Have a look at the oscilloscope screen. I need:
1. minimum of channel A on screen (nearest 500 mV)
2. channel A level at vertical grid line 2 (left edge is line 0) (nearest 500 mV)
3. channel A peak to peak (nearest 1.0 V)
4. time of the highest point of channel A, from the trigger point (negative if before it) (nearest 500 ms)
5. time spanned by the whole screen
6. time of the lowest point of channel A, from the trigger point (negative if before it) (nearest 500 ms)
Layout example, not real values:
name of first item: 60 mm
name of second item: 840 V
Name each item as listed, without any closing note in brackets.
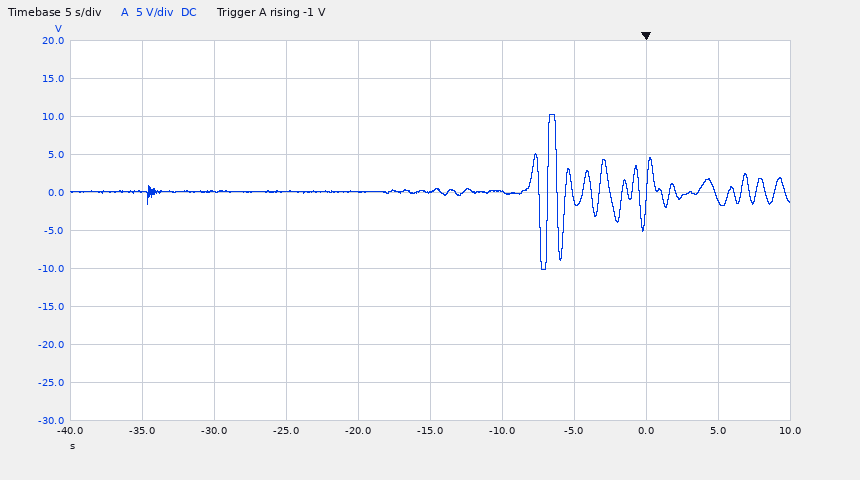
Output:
minimum of channel A on screen: -10.0 V
channel A level at vertical grid line 2 (left edge is line 0): 0.0 V
channel A peak to peak: 20.0 V
time of the highest point of channel A, from the trigger point (negative if before it): -6.5 s
time spanned by the whole screen: 50 s
time of the lowest point of channel A, from the trigger point (negative if before it): -7.0 s
